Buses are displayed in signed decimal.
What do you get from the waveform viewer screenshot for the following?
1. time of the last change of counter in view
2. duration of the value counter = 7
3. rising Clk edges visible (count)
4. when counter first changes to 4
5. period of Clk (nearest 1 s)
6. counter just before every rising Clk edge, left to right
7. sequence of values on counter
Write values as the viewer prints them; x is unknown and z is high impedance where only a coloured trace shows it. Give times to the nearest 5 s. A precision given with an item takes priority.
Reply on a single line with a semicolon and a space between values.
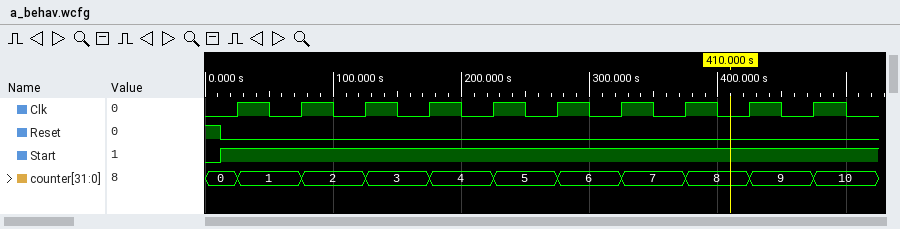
475 s; 50 s; 10; 175 s; 50 s; 0, 1, 2, 3, 4, 5, 6, 7, 8, 9; 0, 1, 2, 3, 4, 5, 6, 7, 8, 9, 10
